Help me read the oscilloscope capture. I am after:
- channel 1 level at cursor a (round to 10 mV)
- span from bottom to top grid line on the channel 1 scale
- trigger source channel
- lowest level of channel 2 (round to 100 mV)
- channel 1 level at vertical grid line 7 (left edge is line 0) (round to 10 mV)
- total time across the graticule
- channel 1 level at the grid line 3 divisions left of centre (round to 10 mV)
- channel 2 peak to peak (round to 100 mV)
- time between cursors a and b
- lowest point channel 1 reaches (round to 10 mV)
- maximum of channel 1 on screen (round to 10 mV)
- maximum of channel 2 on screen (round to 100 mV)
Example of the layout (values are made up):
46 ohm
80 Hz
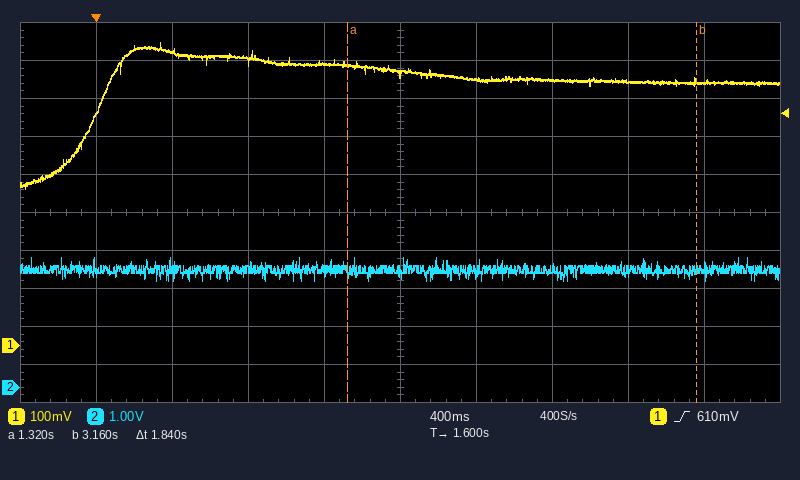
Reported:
740 mV
1 V
channel 1
2.8 V
700 mV
4 s
770 mV
600 mV
1.84 s
410 mV
800 mV
3.4 V
